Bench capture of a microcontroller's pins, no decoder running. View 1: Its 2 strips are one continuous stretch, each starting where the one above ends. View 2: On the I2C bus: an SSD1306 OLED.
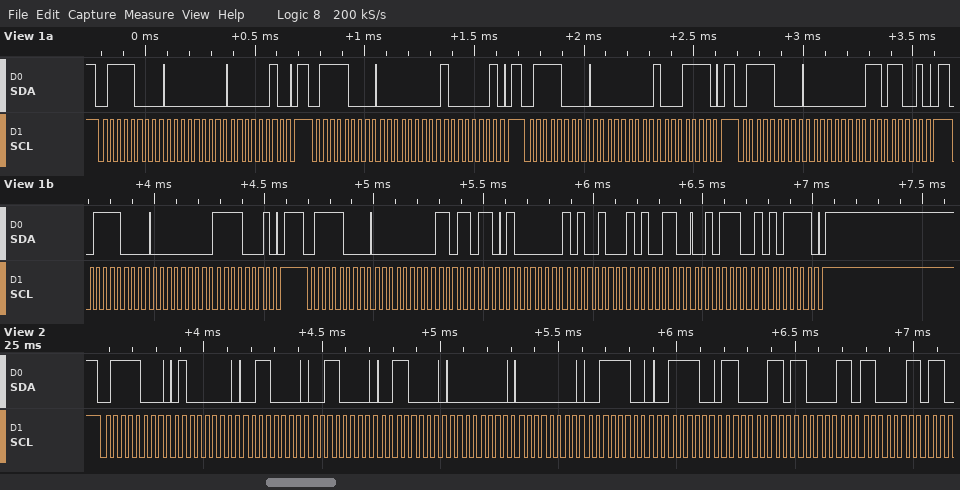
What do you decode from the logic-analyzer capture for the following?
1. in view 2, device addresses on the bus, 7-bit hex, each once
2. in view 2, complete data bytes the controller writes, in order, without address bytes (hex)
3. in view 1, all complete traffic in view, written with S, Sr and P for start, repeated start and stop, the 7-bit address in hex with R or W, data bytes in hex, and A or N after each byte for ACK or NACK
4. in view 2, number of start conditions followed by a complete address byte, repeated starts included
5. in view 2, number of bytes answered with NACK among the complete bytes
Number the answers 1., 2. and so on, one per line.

1. 0x3C
2. 40 30 30 30 00 00 3C 3C C3 C3 C3
3. S 3CW A 00 A 02 A P S 3CW A 00 A 81 A P S 3CW A 00 A 8F A P S 3CW A 00 A D9 A P S 3CW A 00 A F1 A P S 3CW A 00 A DB A 40 A A4 A A6 A 2E A AF A P
4. 1
5. 0
